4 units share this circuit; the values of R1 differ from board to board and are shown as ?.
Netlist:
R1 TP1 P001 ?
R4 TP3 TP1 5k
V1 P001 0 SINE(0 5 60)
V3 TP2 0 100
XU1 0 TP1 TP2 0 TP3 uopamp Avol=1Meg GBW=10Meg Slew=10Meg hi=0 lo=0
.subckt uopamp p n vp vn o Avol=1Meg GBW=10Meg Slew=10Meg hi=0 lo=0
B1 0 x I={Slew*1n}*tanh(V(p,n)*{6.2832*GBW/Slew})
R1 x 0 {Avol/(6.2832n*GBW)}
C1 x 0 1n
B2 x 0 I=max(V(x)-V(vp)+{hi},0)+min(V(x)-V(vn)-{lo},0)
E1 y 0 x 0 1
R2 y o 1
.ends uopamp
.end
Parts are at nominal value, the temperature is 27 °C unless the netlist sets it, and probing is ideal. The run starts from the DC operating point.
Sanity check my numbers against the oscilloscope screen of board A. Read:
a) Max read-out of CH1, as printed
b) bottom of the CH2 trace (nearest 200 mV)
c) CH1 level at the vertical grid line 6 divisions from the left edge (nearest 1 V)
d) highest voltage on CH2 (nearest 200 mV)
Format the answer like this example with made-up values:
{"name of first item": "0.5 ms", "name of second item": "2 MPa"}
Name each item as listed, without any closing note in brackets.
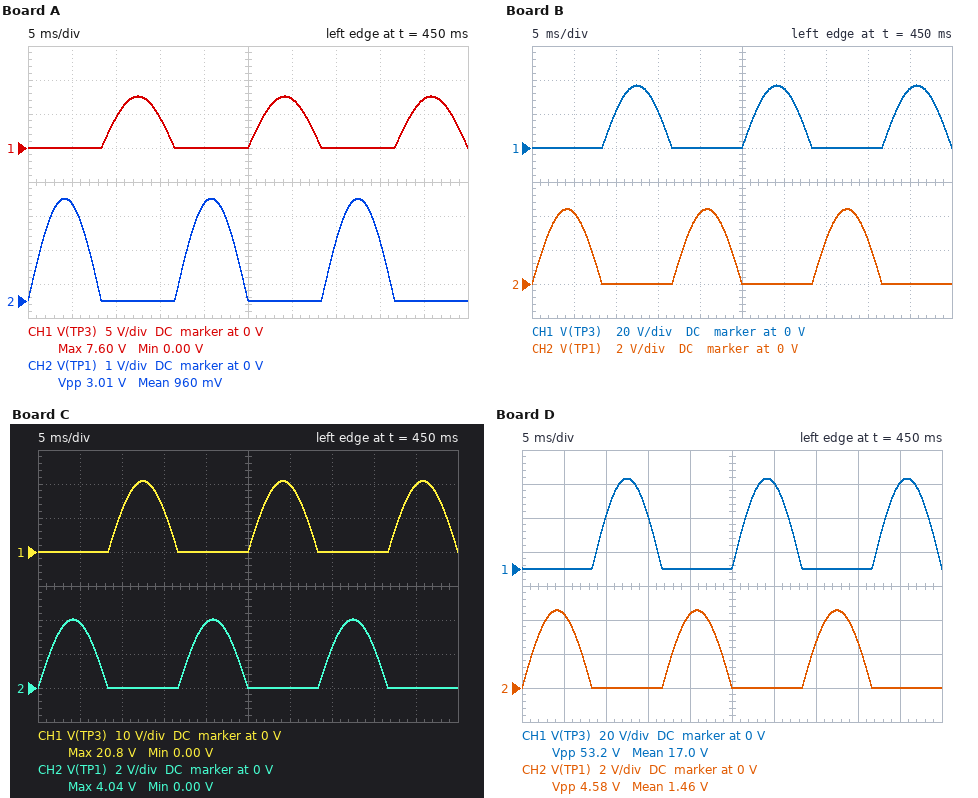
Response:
{"Max read-out of CH1, as printed": "7.60 V", "bottom of the CH2 trace": "0 V", "CH1 level at the vertical grid line 6 divisions from the left edge": "7 V", "highest voltage on CH2": "3.0 V"}
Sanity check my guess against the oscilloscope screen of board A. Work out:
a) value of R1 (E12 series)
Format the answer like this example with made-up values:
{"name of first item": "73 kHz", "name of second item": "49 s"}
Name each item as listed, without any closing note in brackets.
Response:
{"value of R1": "3.3 kΩ"}
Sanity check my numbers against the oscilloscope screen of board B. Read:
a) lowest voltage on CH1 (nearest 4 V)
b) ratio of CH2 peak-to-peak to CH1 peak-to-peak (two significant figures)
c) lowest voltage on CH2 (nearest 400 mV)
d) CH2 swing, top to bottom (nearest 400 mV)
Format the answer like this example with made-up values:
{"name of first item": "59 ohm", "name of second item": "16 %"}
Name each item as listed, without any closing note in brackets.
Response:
{"lowest voltage on CH1": "0 V", "ratio of CH2 peak-to-peak to CH1 peak-to-peak": "0.12", "lowest voltage on CH2": "0 V", "CH2 swing, top to bottom": "4.4 V"}
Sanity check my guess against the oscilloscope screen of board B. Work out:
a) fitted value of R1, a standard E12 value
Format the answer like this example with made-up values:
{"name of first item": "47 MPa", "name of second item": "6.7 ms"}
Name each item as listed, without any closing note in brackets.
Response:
{"fitted value of R1, a standard E12 value": "680 Ω"}
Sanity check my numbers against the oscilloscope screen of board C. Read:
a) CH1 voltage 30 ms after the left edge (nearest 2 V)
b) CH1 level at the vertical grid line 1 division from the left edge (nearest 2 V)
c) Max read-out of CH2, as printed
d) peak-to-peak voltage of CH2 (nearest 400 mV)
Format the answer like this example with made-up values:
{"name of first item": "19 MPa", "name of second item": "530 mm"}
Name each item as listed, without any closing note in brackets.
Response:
{"CH1 voltage 30 ms after the left edge": "20 V", "CH1 level at the vertical grid line 1 division from the left edge": "0 V", "Max read-out of CH2, as printed": "4.04 V", "peak-to-peak voltage of CH2": "4.0 V"}
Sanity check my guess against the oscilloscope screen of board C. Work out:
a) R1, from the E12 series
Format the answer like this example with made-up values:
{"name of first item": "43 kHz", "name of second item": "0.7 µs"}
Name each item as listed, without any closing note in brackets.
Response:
{"R1, from the E12 series": "1.2 kΩ"}
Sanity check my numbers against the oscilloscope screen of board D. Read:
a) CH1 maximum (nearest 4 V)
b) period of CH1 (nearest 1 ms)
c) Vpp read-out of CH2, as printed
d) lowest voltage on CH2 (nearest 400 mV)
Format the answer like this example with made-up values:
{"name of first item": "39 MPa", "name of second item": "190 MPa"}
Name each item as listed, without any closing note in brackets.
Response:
{"CH1 maximum": "52 V", "period of CH1": "17 ms", "Vpp read-out of CH2, as printed": "4.58 V", "lowest voltage on CH2": "0 V"}
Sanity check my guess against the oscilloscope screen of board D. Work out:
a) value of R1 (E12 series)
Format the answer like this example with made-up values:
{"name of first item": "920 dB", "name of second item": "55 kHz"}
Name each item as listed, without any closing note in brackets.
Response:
{"value of R1": "470 Ω"}
